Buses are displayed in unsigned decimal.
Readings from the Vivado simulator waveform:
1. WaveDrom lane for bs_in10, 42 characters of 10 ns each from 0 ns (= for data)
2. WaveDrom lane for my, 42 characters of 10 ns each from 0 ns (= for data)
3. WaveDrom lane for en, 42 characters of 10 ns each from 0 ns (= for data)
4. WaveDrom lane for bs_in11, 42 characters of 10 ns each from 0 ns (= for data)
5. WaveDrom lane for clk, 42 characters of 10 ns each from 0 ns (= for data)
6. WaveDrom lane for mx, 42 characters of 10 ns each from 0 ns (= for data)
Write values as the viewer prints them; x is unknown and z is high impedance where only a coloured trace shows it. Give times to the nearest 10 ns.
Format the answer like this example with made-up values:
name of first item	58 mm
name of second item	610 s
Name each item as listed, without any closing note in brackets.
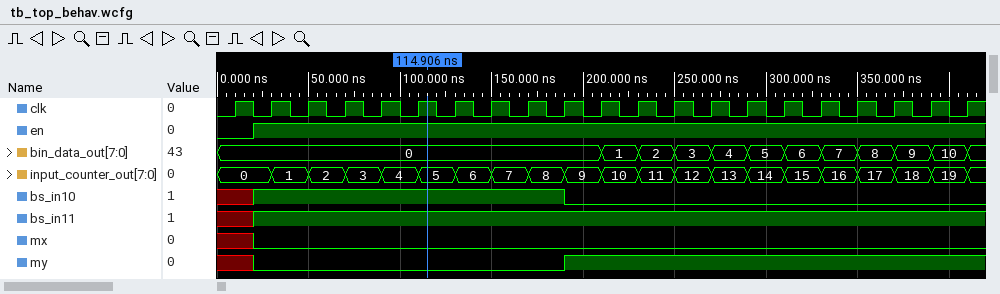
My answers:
WaveDrom lane for bs_in10, 42 characters of 10 ns each from 0 ns	{name: 'bs_in10', wave: 'x.1................0......................'}
WaveDrom lane for my, 42 characters of 10 ns each from 0 ns	{name: 'my', wave: 'x.0................1......................'}
WaveDrom lane for en, 42 characters of 10 ns each from 0 ns	{name: 'en', wave: '0.1.......................................'}
WaveDrom lane for bs_in11, 42 characters of 10 ns each from 0 ns	{name: 'bs_in11', wave: 'x.1.......................................'}
WaveDrom lane for clk, 42 characters of 10 ns each from 0 ns	{name: 'clk', wave: '010101010101010101010101010101010101010101'}
WaveDrom lane for mx, 42 characters of 10 ns each from 0 ns	{name: 'mx', wave: 'x.0.......................................'}
